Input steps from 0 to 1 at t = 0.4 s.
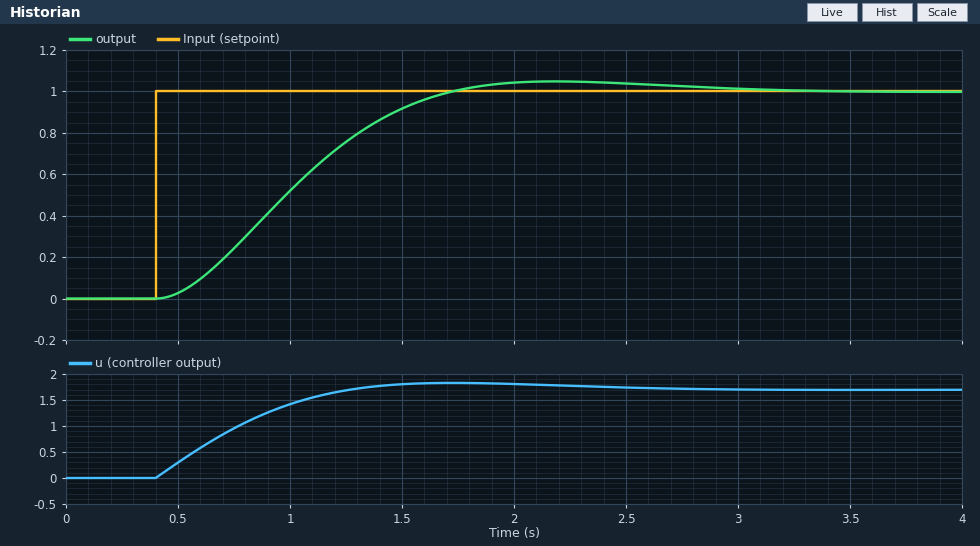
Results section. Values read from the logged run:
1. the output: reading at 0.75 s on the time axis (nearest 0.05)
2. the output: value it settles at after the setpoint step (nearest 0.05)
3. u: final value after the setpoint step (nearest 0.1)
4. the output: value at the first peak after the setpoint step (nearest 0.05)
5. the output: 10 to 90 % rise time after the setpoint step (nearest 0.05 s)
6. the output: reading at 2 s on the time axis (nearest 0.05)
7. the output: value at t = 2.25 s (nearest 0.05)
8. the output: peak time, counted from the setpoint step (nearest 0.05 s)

0.25
1.00
1.7
1.05
0.85 s
1.05
1.05
1.80 s
